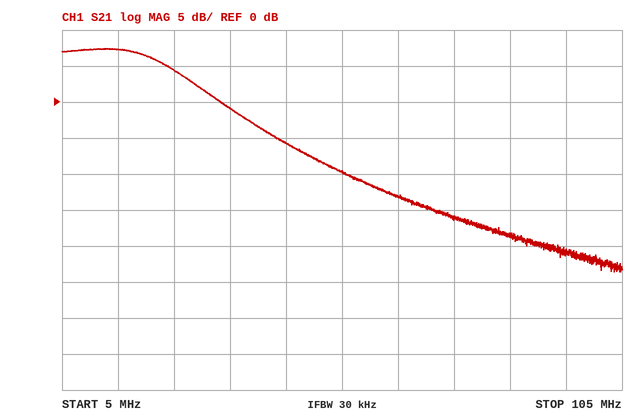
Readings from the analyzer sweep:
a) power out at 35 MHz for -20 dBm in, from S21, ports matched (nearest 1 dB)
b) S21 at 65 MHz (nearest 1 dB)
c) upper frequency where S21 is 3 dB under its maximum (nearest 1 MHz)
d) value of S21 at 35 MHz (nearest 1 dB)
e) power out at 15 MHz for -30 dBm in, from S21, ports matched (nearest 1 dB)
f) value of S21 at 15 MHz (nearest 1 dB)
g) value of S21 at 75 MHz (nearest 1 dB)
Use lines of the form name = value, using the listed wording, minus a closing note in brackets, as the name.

power out at 35 MHz for -20 dBm in, from S21, ports matched = -21 dBm
S21 at 65 MHz = -13 dB
upper frequency where S21 is 3 dB under its maximum = 25 MHz
value of S21 at 35 MHz = -1 dB
power out at 15 MHz for -30 dBm in, from S21, ports matched = -23 dBm
value of S21 at 15 MHz = 7 dB
value of S21 at 75 MHz = -16 dB
